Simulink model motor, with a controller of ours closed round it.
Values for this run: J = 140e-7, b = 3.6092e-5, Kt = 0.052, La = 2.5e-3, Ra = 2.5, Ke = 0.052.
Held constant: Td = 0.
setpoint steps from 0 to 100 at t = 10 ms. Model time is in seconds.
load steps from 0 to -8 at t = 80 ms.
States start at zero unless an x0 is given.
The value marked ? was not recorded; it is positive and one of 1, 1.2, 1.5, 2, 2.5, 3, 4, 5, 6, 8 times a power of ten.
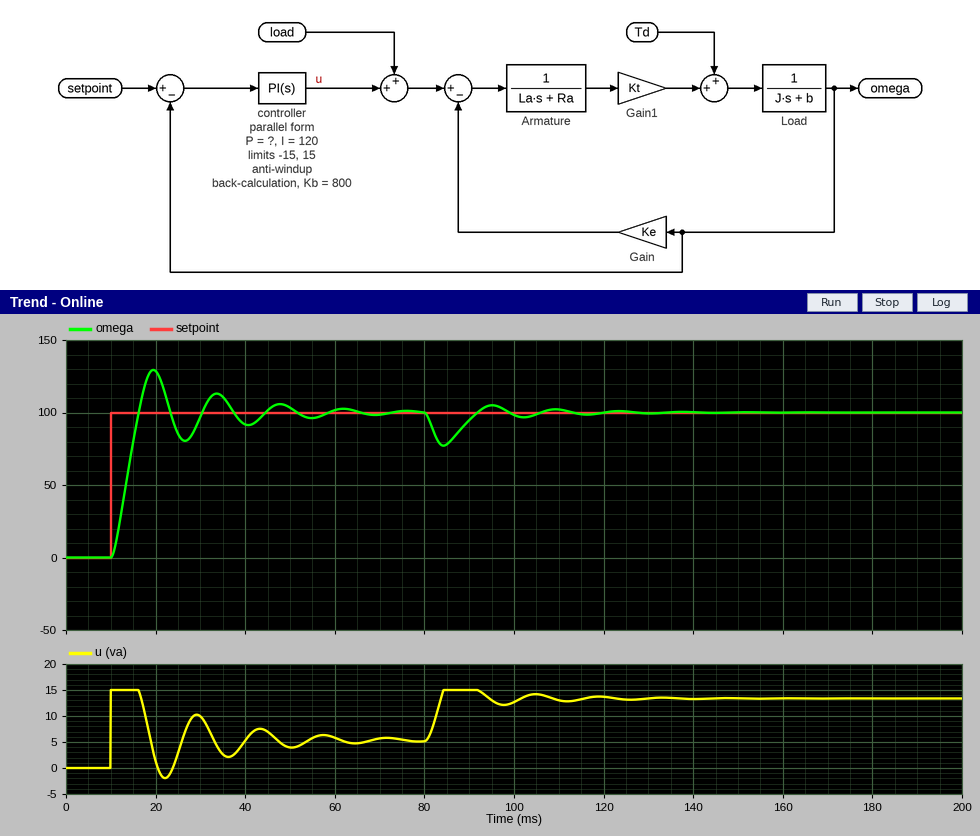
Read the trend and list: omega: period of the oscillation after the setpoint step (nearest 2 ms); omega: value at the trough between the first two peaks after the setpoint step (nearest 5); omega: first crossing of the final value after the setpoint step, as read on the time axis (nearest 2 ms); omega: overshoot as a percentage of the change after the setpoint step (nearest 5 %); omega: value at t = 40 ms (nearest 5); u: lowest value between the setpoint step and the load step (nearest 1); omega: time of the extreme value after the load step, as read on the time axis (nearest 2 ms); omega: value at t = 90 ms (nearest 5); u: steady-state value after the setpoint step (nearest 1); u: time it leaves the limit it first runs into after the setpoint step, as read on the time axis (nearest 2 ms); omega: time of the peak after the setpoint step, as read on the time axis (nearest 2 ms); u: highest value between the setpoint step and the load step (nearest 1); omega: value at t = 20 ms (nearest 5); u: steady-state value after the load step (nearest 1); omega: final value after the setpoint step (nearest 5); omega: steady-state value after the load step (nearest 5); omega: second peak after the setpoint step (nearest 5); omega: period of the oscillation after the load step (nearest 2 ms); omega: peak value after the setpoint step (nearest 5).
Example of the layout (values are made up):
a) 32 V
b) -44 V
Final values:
a) 14 ms
b) 80
c) 16 ms
d) 30 %
e) 90
f) -2
g) 84 ms
h) 95
i) 5
j) 16 ms
k) 20 ms
l) 15
m) 130
n) 13
o) 100
p) 100
q) 115
r) 18 ms
s) 130
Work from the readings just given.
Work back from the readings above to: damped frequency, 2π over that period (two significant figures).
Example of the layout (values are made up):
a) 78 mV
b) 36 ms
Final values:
a) 0.45 rad/ms
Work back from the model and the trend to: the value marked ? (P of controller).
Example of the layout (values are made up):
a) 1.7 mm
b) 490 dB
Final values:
a) 0.15
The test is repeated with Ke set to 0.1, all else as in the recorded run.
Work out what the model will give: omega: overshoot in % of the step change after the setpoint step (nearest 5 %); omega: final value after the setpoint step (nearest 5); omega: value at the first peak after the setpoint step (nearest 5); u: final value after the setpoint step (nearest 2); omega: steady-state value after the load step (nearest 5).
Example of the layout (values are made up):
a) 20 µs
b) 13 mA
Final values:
a) 15 %
b) 100
c) 115
d) 10
e) 70
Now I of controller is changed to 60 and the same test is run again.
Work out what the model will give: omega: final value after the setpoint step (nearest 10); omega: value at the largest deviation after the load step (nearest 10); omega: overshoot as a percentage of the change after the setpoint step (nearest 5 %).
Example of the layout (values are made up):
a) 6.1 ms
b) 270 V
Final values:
a) 100
b) 70
c) 25 %
